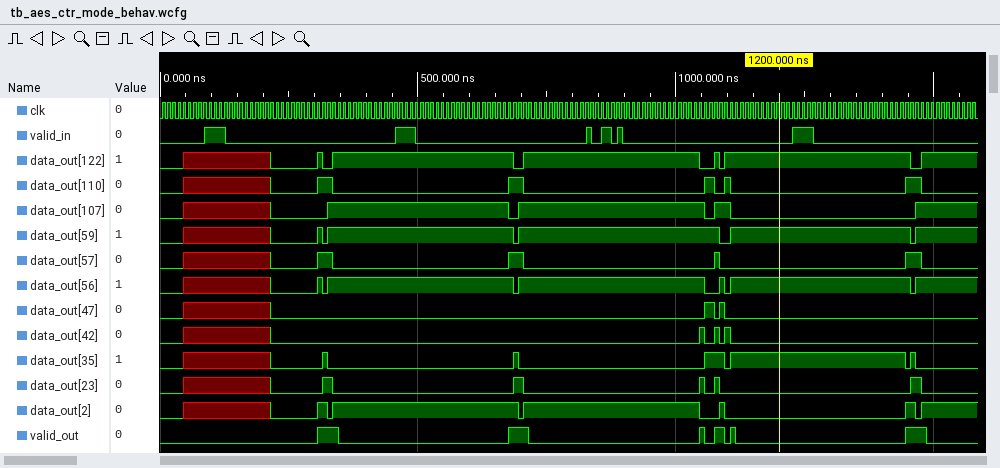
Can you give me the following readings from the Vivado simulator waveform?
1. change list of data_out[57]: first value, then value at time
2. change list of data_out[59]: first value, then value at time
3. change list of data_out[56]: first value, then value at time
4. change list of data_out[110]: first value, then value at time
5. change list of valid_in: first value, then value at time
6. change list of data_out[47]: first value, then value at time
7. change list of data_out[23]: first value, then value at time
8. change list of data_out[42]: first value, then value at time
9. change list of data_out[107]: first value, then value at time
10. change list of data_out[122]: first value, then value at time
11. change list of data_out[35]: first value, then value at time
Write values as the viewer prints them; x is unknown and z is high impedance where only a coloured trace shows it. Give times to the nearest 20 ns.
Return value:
0, x at 40 ns, 0 at 220 ns, 1 at 300 ns, 0 at 340 ns, 1 at 680 ns, 0 at 700 ns, 1 at 1080 ns, 0 at 1080 ns, 1 at 1440 ns, 0 at 1480 ns
0, x at 40 ns, 0 at 220 ns, 1 at 300 ns, 0 at 320 ns, 1 at 320 ns, 0 at 680 ns, 1 at 700 ns, 0 at 1080 ns, 1 at 1100 ns, 0 at 1460 ns, 1 at 1460 ns
0, x at 40 ns, 0 at 220 ns, 1 at 300 ns, 0 at 320 ns, 1 at 320 ns, 0 at 680 ns, 1 at 700 ns, 0 at 1060 ns, 1 at 1080 ns, 0 at 1100 ns, 1 at 1100 ns, 0 at 1460 ns, 1 at 1460 ns
0, x at 40 ns, 0 at 220 ns, 1 at 300 ns, 0 at 340 ns, 1 at 680 ns, 0 at 700 ns, 1 at 1060 ns, 0 at 1080 ns, 1 at 1100 ns, 0 at 1100 ns, 1 at 1440 ns, 0 at 1480 ns
0, 1 at 80 ns, 0 at 120 ns, 1 at 460 ns, 0 at 500 ns, 1 at 820 ns, 0 at 840 ns, 1 at 860 ns, 0 at 880 ns, 1 at 880 ns, 0 at 900 ns, 1 at 1220 ns, 0 at 1260 ns
0, x at 40 ns, 0 at 220 ns, 1 at 1060 ns, 0 at 1080 ns, 1 at 1080 ns, 0 at 1100 ns
0, x at 40 ns, 0 at 220 ns, 1 at 320 ns, 0 at 340 ns, 1 at 680 ns, 0 at 700 ns, 1 at 1040 ns, 0 at 1060 ns, 1 at 1080 ns, 0 at 1080 ns, 1 at 1460 ns, 0 at 1480 ns
0, x at 40 ns, 0 at 220 ns, 1 at 1040 ns, 0 at 1060 ns, 1 at 1080 ns, 0 at 1080 ns, 1 at 1100 ns, 0 at 1100 ns
0, x at 40 ns, 0 at 220 ns, 1 at 320 ns, 0 at 680 ns, 1 at 700 ns, 0 at 1060 ns, 1 at 1080 ns, 0 at 1100 ns, 1 at 1460 ns
0, x at 40 ns, 0 at 220 ns, 1 at 300 ns, 0 at 320 ns, 1 at 340 ns, 0 at 680 ns, 1 at 700 ns, 0 at 1040 ns, 1 at 1080 ns, 0 at 1080 ns, 1 at 1100 ns, 0 at 1460 ns, 1 at 1480 ns
0, x at 40 ns, 0 at 220 ns, 1 at 320 ns, 0 at 320 ns, 1 at 680 ns, 0 at 700 ns, 1 at 1060 ns, 0 at 1100 ns, 1 at 1100 ns, 0 at 1440 ns, 1 at 1460 ns, 0 at 1460 ns
